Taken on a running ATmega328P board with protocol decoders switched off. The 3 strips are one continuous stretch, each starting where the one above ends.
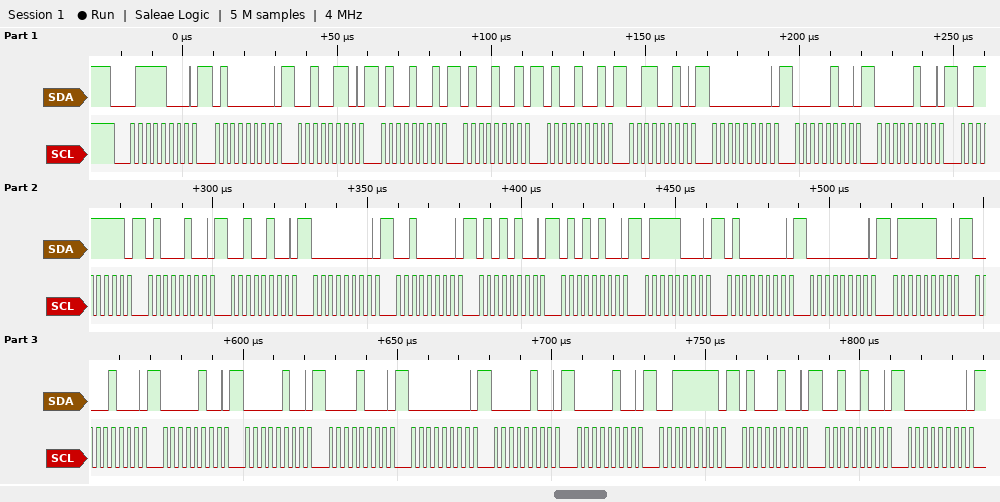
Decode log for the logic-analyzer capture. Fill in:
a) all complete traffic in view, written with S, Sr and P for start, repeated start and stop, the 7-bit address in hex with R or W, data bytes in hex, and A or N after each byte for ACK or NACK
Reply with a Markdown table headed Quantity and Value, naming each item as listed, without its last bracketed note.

| Quantity | Value |
|---|---|
| all complete traffic in view, written with S, Sr and P for start, repeated start and stop, the 7-bit address in hex with R or W, data bytes in hex, and A or N after each byte for ACK or NACK | S 3CW A 40 A 26 A 49 A 49 A 49 A 32 A 00 A 04 A 04 A 3F A 44 A 24 A 00 A 20 A 54 A 54 A 78 A 40 A 00 A 7C A 08 A 04 A 04 A 08 A 00 A 04 A 04 A 3F A 44 A 24 A 00 A |
